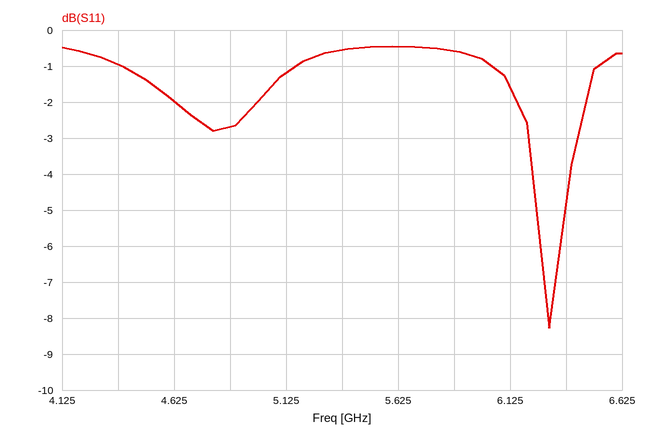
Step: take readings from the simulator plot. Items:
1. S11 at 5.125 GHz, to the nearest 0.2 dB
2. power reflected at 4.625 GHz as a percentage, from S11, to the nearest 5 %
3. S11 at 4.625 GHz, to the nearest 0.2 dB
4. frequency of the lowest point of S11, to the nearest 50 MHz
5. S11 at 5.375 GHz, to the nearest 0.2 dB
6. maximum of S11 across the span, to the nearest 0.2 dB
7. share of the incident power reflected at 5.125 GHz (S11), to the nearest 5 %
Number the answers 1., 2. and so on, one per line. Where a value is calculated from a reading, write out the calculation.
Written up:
1. -1.2 dB
2. 10^(-2/10) ≈ 63.1 %, so 65 % to the nearest 5 %
3. -2.0 dB
4. 6.30 GHz
5. -0.6 dB
6. -0.4 dB
7. 10^(-1.2/10) ≈ 75.9 %, so 75 % to the nearest 5 %
